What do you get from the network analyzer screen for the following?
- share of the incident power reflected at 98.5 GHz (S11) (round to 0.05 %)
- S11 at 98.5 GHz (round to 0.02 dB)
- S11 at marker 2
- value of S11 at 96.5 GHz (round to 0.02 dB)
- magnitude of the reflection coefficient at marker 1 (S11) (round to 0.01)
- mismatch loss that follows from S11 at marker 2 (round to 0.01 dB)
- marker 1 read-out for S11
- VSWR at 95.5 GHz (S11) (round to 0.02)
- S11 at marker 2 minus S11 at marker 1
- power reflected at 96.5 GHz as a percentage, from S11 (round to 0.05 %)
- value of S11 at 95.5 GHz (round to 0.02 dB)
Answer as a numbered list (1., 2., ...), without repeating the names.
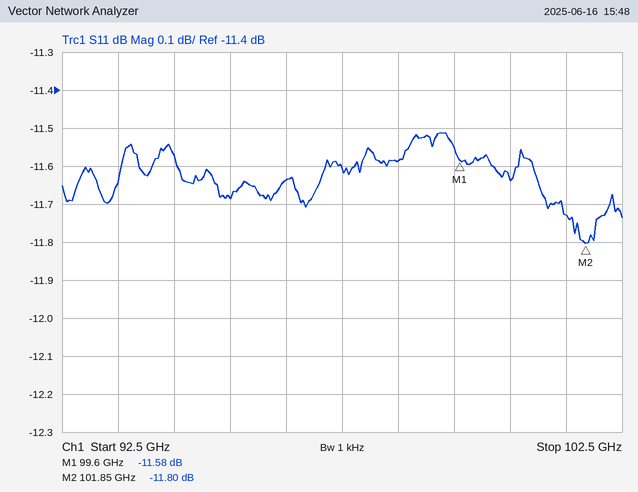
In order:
1. 6.95 %
2. -11.58 dB
3. -11.80 dB
4. -11.64 dB
5. 0.26
6. 0.30 dB
7. -11.58 dB
8. 1.70
9. -0.22 dB
10. 6.85 %
11. -11.68 dB
